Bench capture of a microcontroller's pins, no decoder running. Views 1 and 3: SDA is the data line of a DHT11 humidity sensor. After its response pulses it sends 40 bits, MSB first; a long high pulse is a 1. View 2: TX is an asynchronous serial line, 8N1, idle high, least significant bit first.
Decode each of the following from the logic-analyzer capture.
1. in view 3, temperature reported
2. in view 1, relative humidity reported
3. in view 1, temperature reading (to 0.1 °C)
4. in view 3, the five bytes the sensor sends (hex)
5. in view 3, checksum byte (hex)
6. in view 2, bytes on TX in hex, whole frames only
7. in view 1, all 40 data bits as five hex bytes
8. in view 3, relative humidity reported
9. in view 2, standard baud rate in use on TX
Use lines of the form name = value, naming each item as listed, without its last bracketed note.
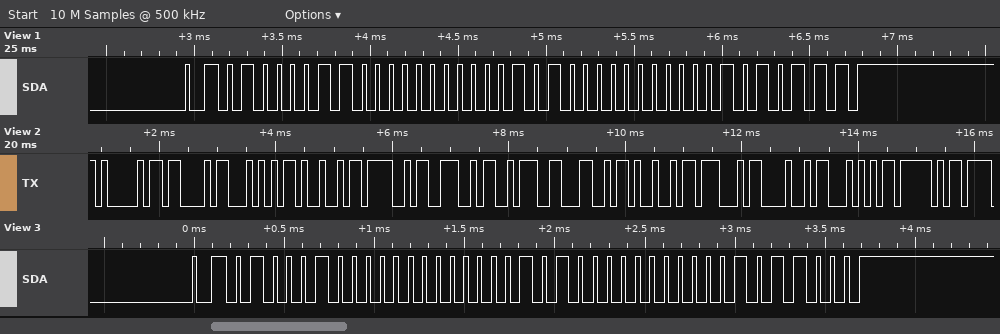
in view 3, temperature reported = 20.0 °C
in view 1, relative humidity reported = 67 %
in view 1, temperature reading = 20.0 °C
in view 3, the five bytes the sensor sends = 44 00 14 00 58
in view 3, checksum byte = 0x58
in view 2, bytes on TX in hex, whole frames only = 0x41 0x43 0x54 0x49 0x4F 0x4E 0x3A 0x4C 0x49 0x47 0x48 0x54 0x5F
in view 1, all 40 data bits as five hex bytes = 43 00 14 00 57
in view 3, relative humidity reported = 68 %
in view 2, standard baud rate in use on TX = 9600 baud
